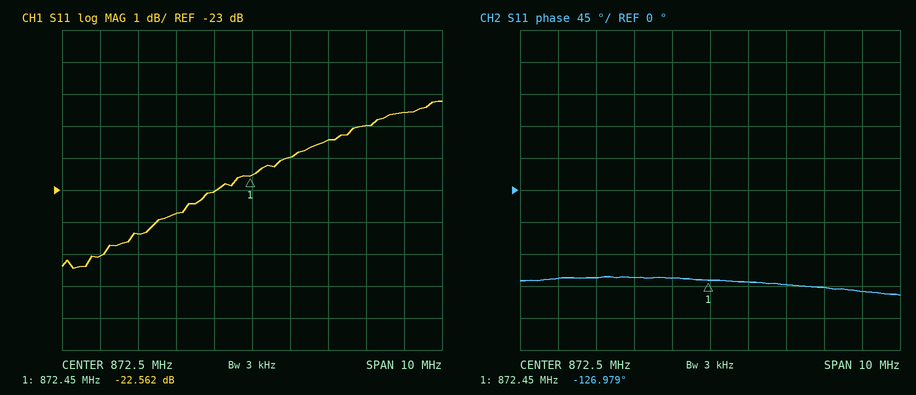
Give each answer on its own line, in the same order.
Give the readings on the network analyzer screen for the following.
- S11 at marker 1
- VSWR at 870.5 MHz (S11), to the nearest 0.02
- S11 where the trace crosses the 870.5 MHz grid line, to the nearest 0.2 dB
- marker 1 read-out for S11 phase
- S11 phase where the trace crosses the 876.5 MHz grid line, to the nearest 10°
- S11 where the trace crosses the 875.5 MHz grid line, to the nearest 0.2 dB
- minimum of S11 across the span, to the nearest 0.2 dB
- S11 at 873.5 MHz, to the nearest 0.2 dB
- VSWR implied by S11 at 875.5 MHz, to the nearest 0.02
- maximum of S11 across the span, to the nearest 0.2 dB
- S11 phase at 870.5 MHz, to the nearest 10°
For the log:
-22.562 dB
1.14
-23.8 dB
-126.979°
-140°
-21.0 dB
-25.4 dB
-22.0 dB
1.20
-20.2 dB
-120°
